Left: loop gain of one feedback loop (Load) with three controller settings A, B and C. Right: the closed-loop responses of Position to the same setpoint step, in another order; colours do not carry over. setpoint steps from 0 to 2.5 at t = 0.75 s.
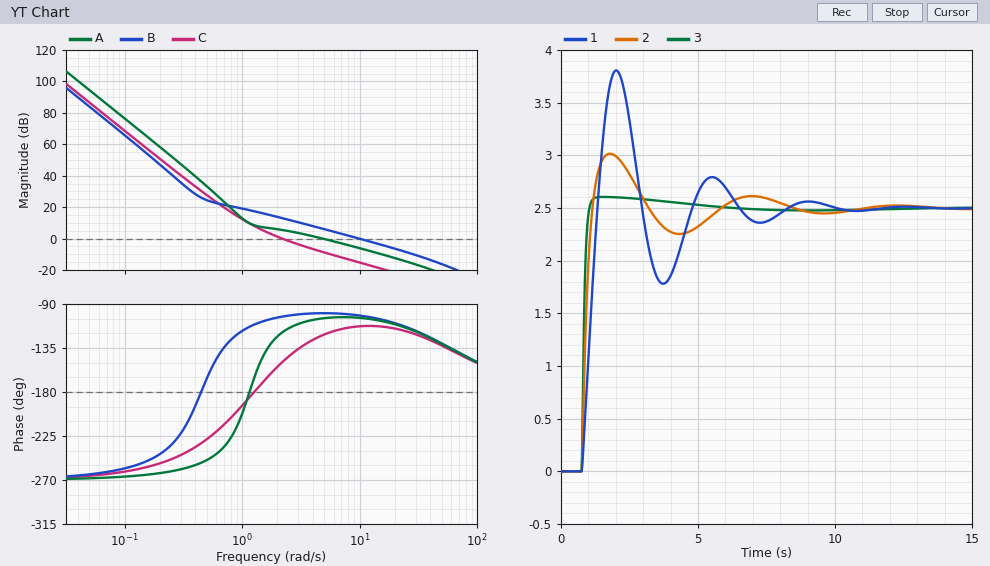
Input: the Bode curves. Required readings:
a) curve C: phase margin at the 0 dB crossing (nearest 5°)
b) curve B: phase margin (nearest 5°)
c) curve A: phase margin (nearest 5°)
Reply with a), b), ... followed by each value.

a) 30°
b) 80°
c) 75°
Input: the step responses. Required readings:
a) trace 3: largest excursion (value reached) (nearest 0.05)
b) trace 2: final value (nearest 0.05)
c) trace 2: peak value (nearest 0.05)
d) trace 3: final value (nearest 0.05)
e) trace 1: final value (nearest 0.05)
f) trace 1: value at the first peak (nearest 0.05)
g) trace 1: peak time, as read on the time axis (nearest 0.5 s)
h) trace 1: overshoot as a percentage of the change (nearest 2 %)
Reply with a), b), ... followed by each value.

a) 2.60
b) 2.50
c) 3.00
d) 2.50
e) 2.50
f) 3.80
g) 2.0 s
h) 52 %
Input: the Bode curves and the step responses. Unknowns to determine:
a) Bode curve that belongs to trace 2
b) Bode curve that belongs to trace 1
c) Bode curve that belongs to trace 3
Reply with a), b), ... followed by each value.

a) A
b) C
c) B
